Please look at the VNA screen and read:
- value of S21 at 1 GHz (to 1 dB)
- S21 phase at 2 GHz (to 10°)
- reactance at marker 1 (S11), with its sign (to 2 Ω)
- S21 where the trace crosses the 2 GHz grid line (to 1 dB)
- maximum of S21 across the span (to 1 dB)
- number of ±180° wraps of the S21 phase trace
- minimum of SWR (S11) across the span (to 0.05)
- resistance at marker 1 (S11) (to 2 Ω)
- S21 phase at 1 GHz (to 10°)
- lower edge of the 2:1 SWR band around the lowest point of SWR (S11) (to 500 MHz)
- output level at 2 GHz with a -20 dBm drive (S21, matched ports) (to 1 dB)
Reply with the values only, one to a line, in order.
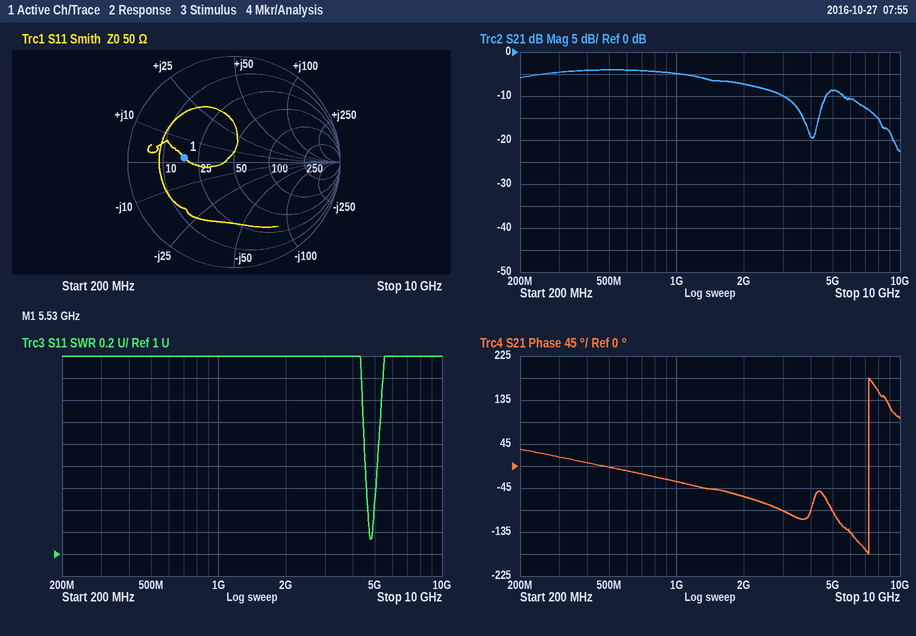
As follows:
-5 dB
-60°
+2 Ω
-7 dB
-4 dB
1
1.15
18 Ω
-30°
4.5 GHz
-27 dBm
